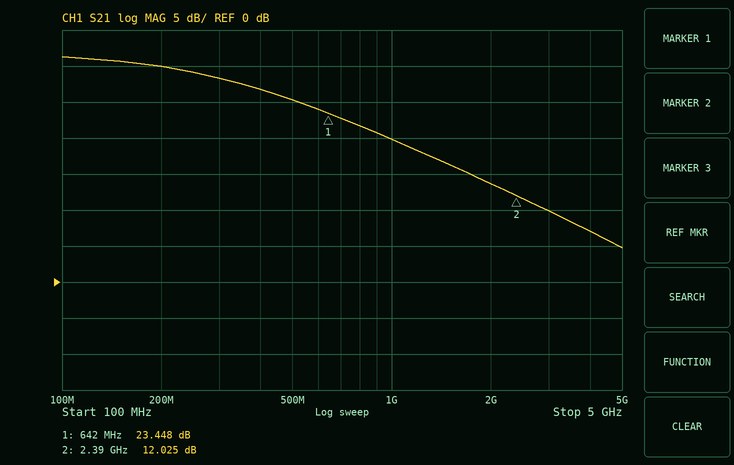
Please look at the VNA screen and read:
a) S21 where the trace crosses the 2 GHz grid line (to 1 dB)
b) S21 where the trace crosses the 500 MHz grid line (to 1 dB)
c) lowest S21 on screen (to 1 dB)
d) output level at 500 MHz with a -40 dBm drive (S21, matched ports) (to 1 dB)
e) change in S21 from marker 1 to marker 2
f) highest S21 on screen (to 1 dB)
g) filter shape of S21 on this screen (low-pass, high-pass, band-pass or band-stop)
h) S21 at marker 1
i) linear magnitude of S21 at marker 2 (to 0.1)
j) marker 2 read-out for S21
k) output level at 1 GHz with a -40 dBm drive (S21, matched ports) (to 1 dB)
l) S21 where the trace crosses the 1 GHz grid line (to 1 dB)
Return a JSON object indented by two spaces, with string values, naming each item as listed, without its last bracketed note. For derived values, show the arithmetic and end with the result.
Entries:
{
  "S21 where the trace crosses the 2 GHz grid line": "14 dB",
  "S21 where the trace crosses the 500 MHz grid line": "25 dB",
  "lowest S21 on screen": "5 dB",
  "output level at 500 MHz with a -40 dBm drive (S21, matched ports)": "-40 dBm + (25 dB) = -15 dBm",
  "change in S21 from marker 1 to marker 2": "12.025 − (23.448) = -11.423 dB",
  "highest S21 on screen": "31 dB",
  "filter shape of S21 on this screen": "low-pass",
  "S21 at marker 1": "23.448 dB",
  "linear magnitude of S21 at marker 2": "10^(12.025/20) ≈ 4.0",
  "marker 2 read-out for S21": "12.025 dB",
  "output level at 1 GHz with a -40 dBm drive (S21, matched ports)": "-40 dBm + (20 dB) = -20 dBm",
  "S21 where the trace crosses the 1 GHz grid line": "20 dB"
}
